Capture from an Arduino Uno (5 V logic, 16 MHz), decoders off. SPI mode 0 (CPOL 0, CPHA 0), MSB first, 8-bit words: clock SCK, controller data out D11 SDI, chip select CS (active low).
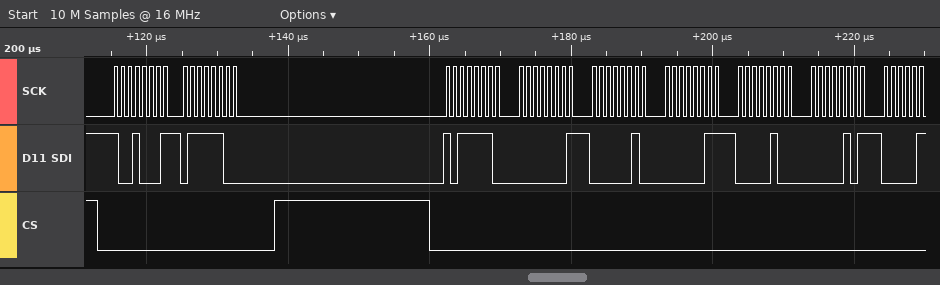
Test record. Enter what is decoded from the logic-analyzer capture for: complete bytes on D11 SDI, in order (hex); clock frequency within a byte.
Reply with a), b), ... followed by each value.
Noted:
a) 91 7C BE 01 02 03 04 05
b) 1 MHz
